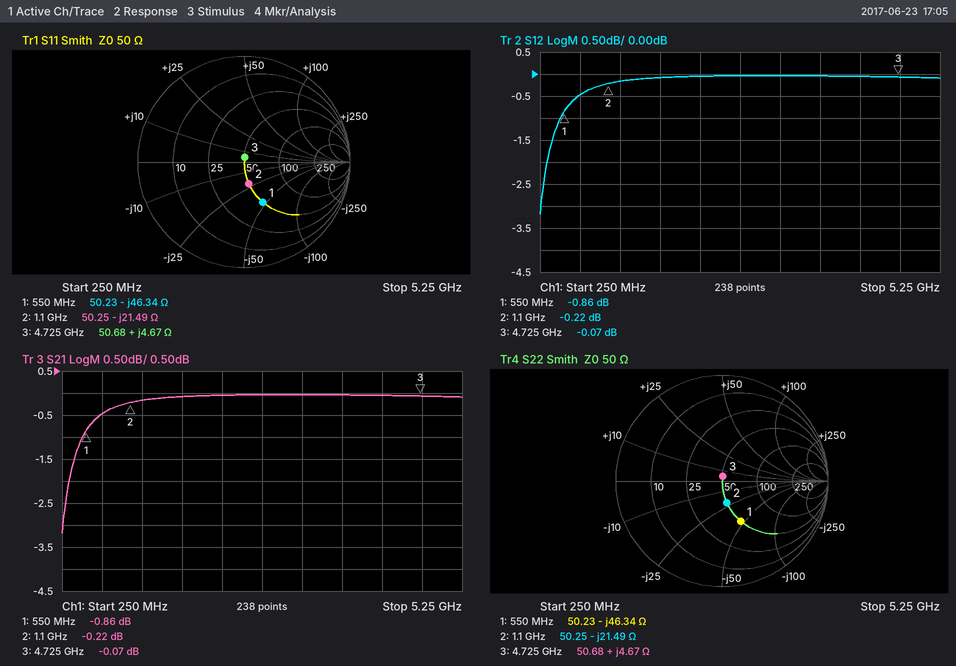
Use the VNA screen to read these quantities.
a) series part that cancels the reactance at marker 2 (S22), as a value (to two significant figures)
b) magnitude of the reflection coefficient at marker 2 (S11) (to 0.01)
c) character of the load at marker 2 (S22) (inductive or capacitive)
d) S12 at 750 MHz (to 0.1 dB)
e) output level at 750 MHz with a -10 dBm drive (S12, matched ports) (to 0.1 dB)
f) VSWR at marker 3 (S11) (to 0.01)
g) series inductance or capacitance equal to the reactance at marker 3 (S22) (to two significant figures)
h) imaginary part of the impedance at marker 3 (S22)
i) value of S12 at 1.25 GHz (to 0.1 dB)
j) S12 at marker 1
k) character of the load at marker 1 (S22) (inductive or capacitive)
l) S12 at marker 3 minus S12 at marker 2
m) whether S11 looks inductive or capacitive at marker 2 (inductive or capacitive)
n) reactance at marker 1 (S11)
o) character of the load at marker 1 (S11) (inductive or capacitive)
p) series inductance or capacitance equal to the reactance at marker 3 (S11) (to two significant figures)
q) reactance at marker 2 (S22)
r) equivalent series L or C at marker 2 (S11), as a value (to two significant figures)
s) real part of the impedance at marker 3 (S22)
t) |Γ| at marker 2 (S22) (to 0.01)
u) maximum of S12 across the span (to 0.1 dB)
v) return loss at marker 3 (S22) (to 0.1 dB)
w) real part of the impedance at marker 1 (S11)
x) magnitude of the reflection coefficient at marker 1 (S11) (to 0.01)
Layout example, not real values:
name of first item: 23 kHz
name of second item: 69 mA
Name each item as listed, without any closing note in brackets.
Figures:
series part that cancels the reactance at marker 2 (S22), as a value: 3.1 nH
magnitude of the reflection coefficient at marker 2 (S11): 0.21
character of the load at marker 2 (S22): capacitive
S12 at 750 MHz: -0.5 dB
output level at 750 MHz with a -10 dBm drive (S12, matched ports): -10.5 dBm
VSWR at marker 3 (S11): 1.10
series inductance or capacitance equal to the reactance at marker 3 (S22): 160 pH
imaginary part of the impedance at marker 3: +4.67 Ω
value of S12 at 1.25 GHz: -0.2 dB
S12 at marker 1: -0.86 dB
character of the load at marker 1 (S22): capacitive
S12 at marker 3 minus S12 at marker 2: 0.15 dB
whether S11 looks inductive or capacitive at marker 2: capacitive
reactance at marker 1: -46.34 Ω
character of the load at marker 1 (S11): capacitive
series inductance or capacitance equal to the reactance at marker 3 (S11): 160 pH
reactance at marker 2: -21.49 Ω
equivalent series L or C at marker 2 (S11), as a value: 6.7 pF
real part of the impedance at marker 3: 50.68 Ω
|Γ| at marker 2 (S22): 0.21
maximum of S12 across the span: 0.0 dB
return loss at marker 3 (S22): 26.6 dB
real part of the impedance at marker 1: 50.23 Ω
magnitude of the reflection coefficient at marker 1 (S11): 0.42
